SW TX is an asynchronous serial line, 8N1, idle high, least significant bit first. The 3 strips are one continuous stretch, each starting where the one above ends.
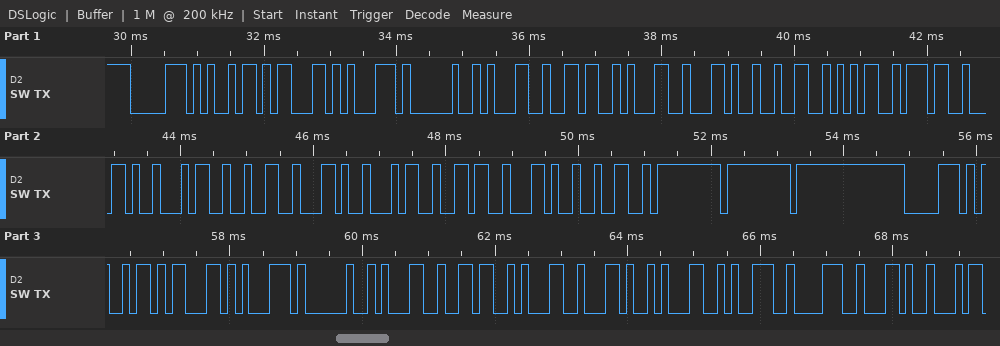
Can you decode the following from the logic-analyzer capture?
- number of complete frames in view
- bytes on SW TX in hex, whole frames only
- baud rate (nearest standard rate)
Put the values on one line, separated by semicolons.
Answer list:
36; 0x70 0x69 0x63 0x71 0x20 0x31 0x36 0x31 0x2C 0x32 0x35 0x37 0x2C 0x34 0x32 0x2C 0x34 0x36 0x2C 0x32 0xFF 0xFF 0xFF 0x70 0x69 0x63 0x71 0x20 0x31 0x36 0x31 0x2C 0x31 0x39 0x38 0x2C; 9600 baud
